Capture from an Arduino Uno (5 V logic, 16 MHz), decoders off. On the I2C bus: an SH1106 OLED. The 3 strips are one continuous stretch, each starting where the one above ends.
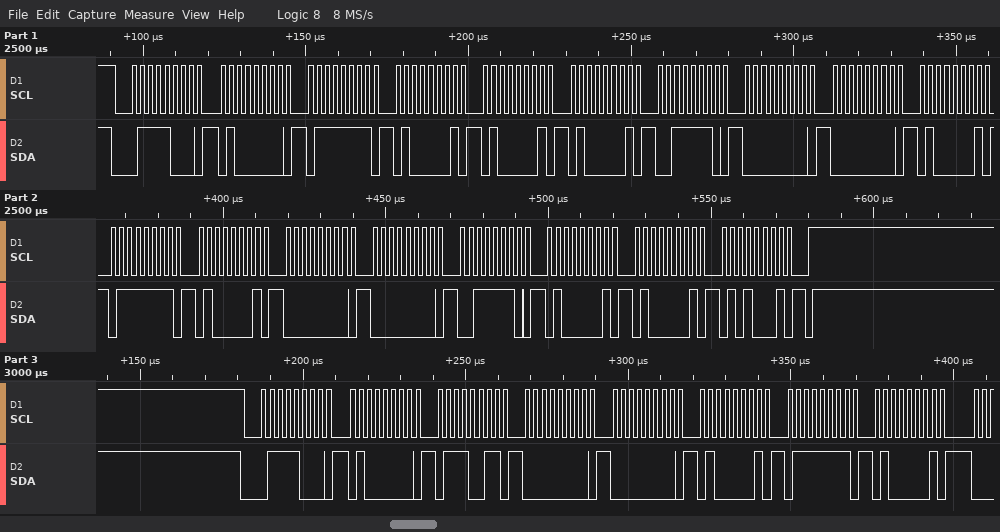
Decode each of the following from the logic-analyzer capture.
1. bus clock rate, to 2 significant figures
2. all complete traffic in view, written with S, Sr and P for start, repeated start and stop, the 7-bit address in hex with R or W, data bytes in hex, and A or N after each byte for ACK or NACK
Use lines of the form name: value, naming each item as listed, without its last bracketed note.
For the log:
bus clock rate, to 2 significant figures: 400 kHz
all complete traffic in view, written with S, Sr and P for start, repeated start and stop, the 7-bit address in hex with R or W, data bytes in hex, and A or N after each byte for ACK or NACK: S 3CW A 40 A 7F A 41 A 41 A 41 A 3E A 00 A 00 A 41 A 7F A 41 A 00 A 00 A 3E A 41 A 41 A 51 A P S 3CW A 40 A 73 A 00 A 00 A 41 A 7F A 41 A
